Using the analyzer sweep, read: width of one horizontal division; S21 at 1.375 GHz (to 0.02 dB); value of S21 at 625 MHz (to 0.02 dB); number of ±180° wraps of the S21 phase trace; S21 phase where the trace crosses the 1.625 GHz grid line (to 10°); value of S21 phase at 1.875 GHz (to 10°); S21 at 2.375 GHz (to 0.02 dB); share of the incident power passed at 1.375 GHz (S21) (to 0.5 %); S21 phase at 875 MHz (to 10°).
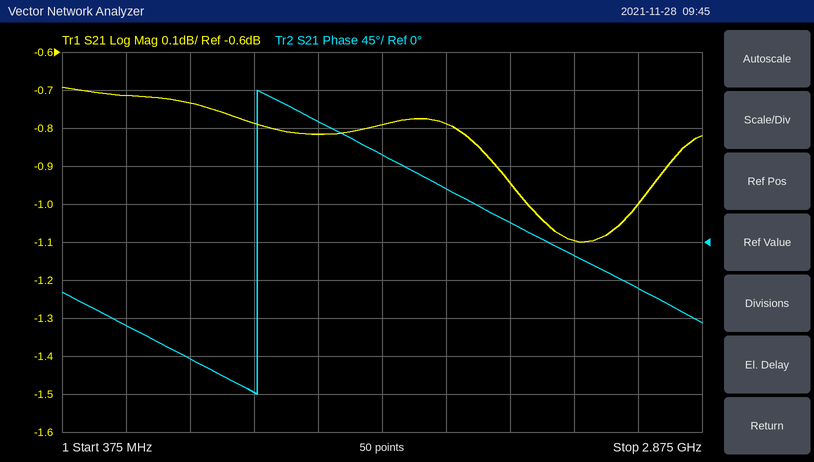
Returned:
250 MHz
-0.82 dB
-0.72 dB
1
100°
60°
-1.10 dB
83.0 %
-140°
